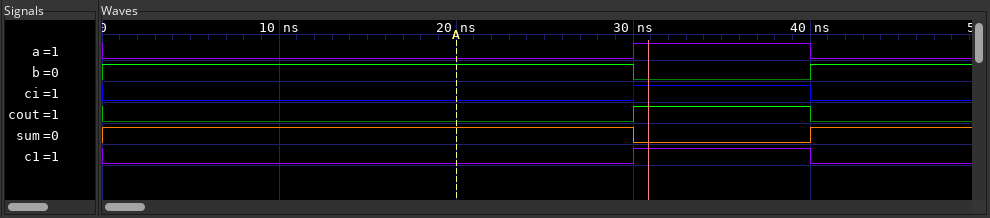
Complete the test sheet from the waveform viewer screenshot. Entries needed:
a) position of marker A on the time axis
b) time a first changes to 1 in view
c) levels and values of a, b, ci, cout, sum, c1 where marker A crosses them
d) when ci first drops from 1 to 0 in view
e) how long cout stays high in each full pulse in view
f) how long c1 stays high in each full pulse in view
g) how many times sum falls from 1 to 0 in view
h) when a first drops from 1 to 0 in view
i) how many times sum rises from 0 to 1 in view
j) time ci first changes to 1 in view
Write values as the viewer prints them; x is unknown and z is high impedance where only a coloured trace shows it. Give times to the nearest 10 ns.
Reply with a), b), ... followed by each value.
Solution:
a) 20 ns
b) 30 ns
c) a=0, b=1, ci=0, cout=0, sum=1, c1=0
d) 40 ns
e) 10 ns
f) 10 ns
g) 1
h) 40 ns
i) 1
j) 30 ns
